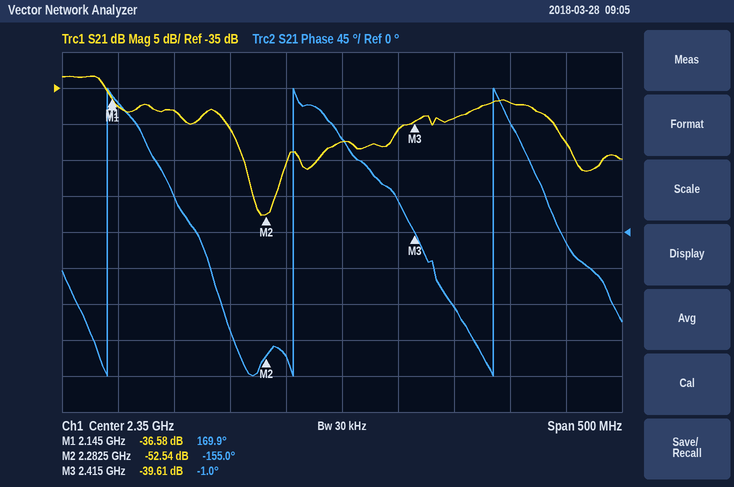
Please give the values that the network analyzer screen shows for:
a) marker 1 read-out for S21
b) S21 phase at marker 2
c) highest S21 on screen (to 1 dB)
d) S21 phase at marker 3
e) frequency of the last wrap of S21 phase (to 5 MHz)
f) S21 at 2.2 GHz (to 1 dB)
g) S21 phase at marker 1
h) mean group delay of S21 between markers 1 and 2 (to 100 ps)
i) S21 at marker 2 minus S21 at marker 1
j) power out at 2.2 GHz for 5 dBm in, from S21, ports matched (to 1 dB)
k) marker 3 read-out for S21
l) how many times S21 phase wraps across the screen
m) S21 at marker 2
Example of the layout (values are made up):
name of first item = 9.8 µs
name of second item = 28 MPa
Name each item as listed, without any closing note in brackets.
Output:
marker 1 read-out for S21 = -36.58 dB
S21 phase at marker 2 = -155.0°
highest S21 on screen = -33 dB
S21 phase at marker 3 = -1.0°
frequency of the last wrap of S21 phase = 2.485 GHz
S21 at 2.2 GHz = -38 dB
S21 phase at marker 1 = 169.9°
mean group delay of S21 between markers 1 and 2 = 6.6 ns
S21 at marker 2 minus S21 at marker 1 = -15.96 dB
power out at 2.2 GHz for 5 dBm in, from S21, ports matched = -33 dBm
marker 3 read-out for S21 = -39.61 dB
how many times S21 phase wraps across the screen = 3
S21 at marker 2 = -52.54 dB
